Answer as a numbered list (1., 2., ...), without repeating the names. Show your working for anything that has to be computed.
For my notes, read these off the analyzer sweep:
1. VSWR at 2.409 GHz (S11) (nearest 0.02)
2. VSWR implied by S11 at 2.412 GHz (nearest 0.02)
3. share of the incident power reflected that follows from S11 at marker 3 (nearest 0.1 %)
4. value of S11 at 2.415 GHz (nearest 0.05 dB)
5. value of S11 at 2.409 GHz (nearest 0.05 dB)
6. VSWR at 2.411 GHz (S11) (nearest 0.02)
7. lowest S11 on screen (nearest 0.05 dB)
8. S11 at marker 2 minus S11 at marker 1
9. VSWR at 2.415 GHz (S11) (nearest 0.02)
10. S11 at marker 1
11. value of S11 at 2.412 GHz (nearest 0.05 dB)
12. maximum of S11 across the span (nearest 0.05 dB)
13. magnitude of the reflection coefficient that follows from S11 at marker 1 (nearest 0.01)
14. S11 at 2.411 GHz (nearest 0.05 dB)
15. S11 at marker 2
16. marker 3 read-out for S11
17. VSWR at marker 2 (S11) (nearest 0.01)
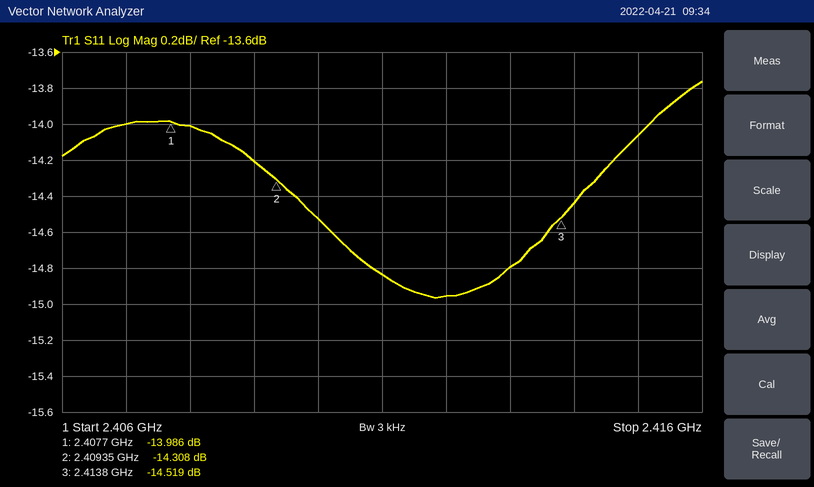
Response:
1. |Γ| = 10^(-14.2/20) = 0.1950; VSWR = (1 + 0.1950)/(1 − 0.1950) ≈ 1.48
2. |Γ| = 10^(-14.95/20) = 0.1789; VSWR = (1 + 0.1789)/(1 − 0.1789) ≈ 1.44
3. 10^(-14.519/10) ≈ 3.5 %
4. -14.05 dB
5. -14.20 dB
6. |Γ| = 10^(-14.85/20) = 0.1809; VSWR = (1 + 0.1809)/(1 − 0.1809) ≈ 1.44
7. -14.95 dB
8. -14.308 − (-13.986) = -0.322 dB
9. |Γ| = 10^(-14.05/20) = 0.1984; VSWR = (1 + 0.1984)/(1 − 0.1984) ≈ 1.49, so 1.50 to the nearest 0.02
10. -13.986 dB
11. -14.95 dB
12. -13.75 dB
13. 10^(-13.986/20) ≈ 0.20
14. -14.85 dB
15. -14.308 dB
16. -14.519 dB
17. (1 + 0.1926)/(1 − 0.1926) ≈ 1.48
